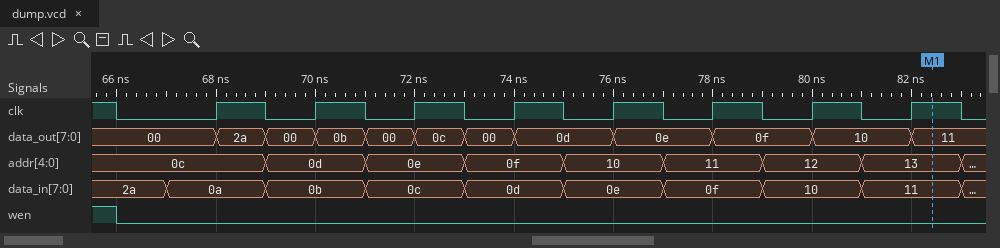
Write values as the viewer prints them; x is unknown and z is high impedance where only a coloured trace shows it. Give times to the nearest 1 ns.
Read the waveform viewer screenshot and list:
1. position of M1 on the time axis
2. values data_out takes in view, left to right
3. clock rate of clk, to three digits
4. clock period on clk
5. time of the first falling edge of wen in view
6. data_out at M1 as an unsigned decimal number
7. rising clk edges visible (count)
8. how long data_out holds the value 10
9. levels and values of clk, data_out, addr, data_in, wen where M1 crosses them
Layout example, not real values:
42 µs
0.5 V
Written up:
82 ns
00, 2a, 00, 0b, 00, 0c, 00, 0d, 0e, 0f, 10, 11
500 MHz
2 ns
66 ns
17
8
2 ns
clk=1, data_out=11, addr=13, data_in=11, wen=0
